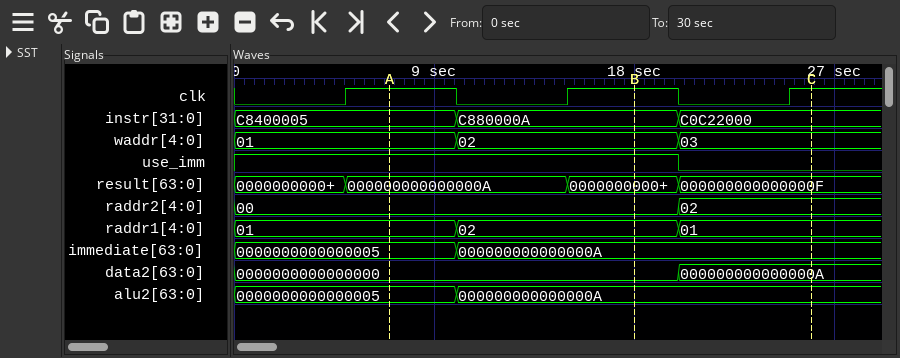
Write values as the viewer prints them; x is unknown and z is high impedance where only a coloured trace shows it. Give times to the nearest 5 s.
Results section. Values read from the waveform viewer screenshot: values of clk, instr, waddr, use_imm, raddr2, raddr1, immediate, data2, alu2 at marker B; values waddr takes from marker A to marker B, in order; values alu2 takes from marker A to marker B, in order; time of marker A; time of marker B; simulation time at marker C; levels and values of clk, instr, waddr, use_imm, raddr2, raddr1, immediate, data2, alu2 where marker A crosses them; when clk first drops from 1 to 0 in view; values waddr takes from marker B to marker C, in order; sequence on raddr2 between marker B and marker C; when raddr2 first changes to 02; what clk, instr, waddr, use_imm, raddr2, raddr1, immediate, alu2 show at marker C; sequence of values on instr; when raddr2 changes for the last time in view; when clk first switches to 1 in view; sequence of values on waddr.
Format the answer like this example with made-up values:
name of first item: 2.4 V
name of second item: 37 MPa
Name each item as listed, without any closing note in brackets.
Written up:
values of clk, instr, waddr, use_imm, raddr2, raddr1, immediate, data2, alu2 at marker B: clk=1, instr=C880000A, waddr=02, use_imm=1, raddr2=00, raddr1=02, immediate=000000000000000A, data2=0000000000000000, alu2=000000000000000A
values waddr takes from marker A to marker B, in order: 01, 02
values alu2 takes from marker A to marker B, in order: 0000000000000005, 000000000000000A
time of marker A: 5 s
time of marker B: 20 s
simulation time at marker C: 25 s
levels and values of clk, instr, waddr, use_imm, raddr2, raddr1, immediate, data2, alu2 where marker A crosses them: clk=1, instr=C8400005, waddr=01, use_imm=1, raddr2=00, raddr1=01, immediate=0000000000000005, data2=0000000000000000, alu2=0000000000000005
when clk first drops from 1 to 0 in view: 10 s
values waddr takes from marker B to marker C, in order: 02, 03
sequence on raddr2 between marker B and marker C: 00, 02
when raddr2 first changes to 02: 20 s
what clk, instr, waddr, use_imm, raddr2, raddr1, immediate, alu2 show at marker C: clk=1, instr=C0C22000, waddr=03, use_imm=0, raddr2=02, raddr1=01, immediate=000000000000000A, alu2=000000000000000A
sequence of values on instr: C8400005, C880000A, C0C22000
when raddr2 changes for the last time in view: 20 s
when clk first switches to 1 in view: 5 s
sequence of values on waddr: 01, 02, 03
